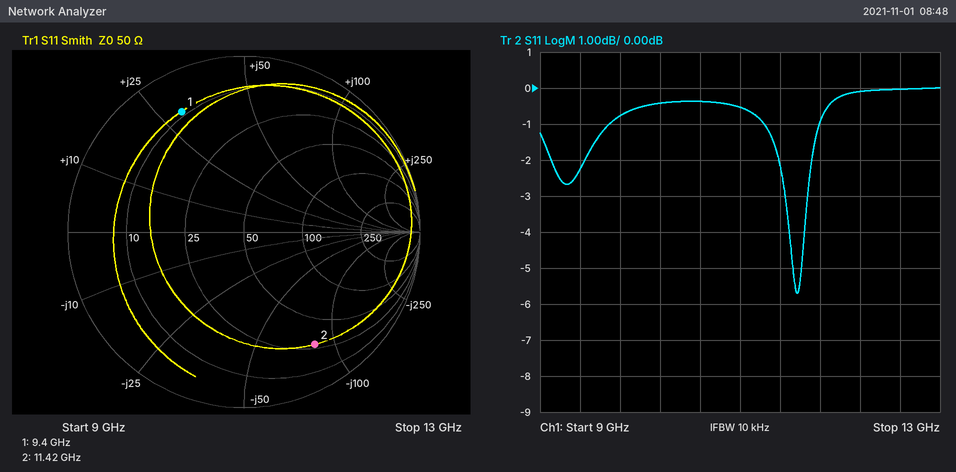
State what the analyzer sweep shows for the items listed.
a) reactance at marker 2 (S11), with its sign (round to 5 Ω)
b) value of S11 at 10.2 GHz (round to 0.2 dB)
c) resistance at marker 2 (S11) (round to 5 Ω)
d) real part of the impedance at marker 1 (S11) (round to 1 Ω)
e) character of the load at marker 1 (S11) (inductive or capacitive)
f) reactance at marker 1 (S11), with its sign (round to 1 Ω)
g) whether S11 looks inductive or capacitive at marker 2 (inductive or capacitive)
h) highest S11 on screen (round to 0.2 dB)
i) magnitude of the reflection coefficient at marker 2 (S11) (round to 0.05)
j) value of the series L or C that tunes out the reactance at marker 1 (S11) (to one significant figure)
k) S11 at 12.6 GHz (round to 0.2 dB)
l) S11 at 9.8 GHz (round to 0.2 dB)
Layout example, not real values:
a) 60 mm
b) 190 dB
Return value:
a) -85 Ω
b) -0.4 dB
c) 30 Ω
d) 9 Ω
e) inductive
f) +30 Ω
g) capacitive
h) 0.0 dB
i) 0.75
j) 600 fF
k) 0.0 dB
l) -0.8 dB
